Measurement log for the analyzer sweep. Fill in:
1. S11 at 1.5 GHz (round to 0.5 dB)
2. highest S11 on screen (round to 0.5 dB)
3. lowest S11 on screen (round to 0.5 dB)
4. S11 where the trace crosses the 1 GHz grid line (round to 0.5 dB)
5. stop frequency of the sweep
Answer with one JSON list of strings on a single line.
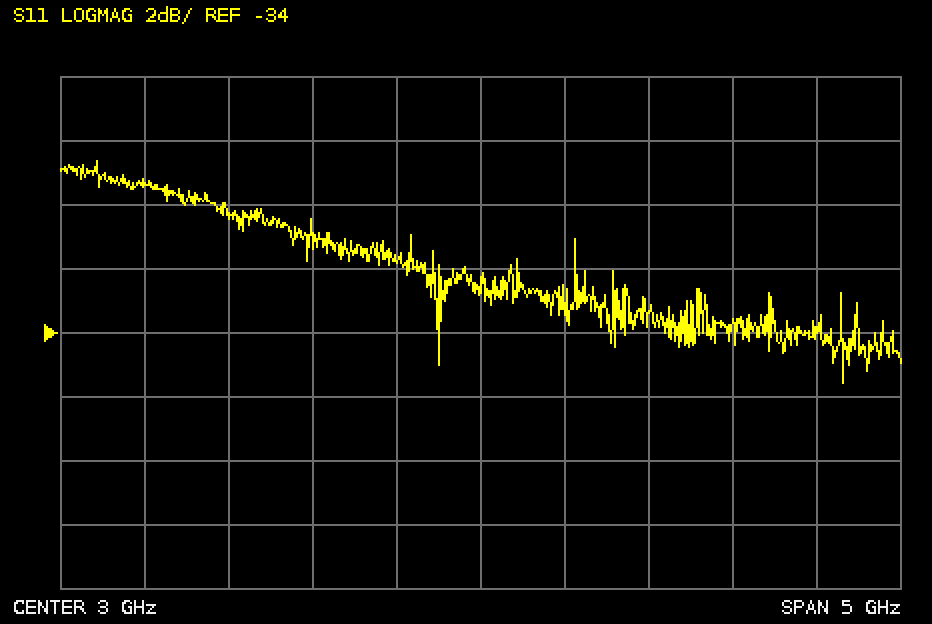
["-30.5 dB", "-28.5 dB", "-35.5 dB", "-29.5 dB", "5.5 GHz"]
